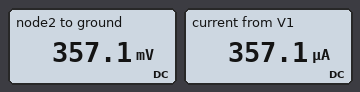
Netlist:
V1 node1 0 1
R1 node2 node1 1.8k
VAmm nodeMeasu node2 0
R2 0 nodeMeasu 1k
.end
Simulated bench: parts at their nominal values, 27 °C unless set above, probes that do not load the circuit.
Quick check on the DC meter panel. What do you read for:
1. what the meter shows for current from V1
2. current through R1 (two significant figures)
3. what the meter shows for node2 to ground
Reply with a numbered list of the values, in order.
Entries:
1. 357.1 µA
2. 360 µA
3. 357.1 mV
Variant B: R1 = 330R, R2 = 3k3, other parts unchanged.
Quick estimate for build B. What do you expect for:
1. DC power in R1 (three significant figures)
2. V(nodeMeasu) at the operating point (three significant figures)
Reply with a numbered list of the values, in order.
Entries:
1. 25.0 µW
2. 909 mV
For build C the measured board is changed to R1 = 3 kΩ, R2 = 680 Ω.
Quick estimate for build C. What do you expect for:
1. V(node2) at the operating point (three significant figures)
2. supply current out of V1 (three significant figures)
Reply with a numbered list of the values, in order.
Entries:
1. 185 mV
2. 272 µA
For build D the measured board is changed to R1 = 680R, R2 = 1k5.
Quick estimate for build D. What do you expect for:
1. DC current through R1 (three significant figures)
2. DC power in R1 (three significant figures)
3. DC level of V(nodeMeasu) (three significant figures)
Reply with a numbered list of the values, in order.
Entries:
1. 459 µA
2. 143 µW
3. 688 mV
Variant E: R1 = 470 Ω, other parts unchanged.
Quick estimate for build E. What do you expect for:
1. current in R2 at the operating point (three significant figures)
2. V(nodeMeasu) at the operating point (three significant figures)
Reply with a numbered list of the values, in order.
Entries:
1. 680 µA
2. 680 mV
